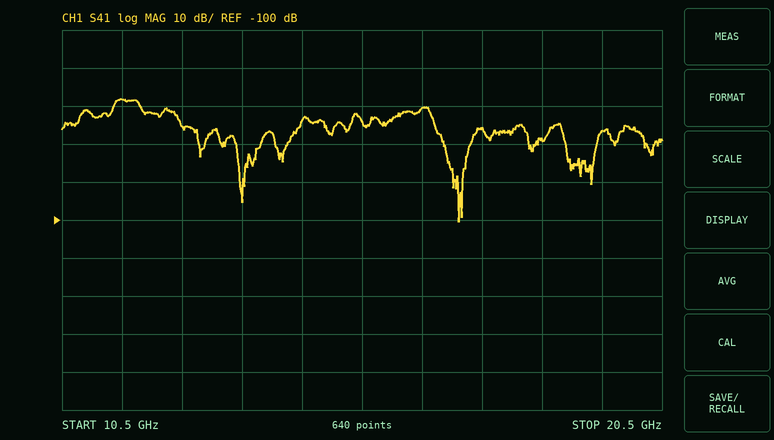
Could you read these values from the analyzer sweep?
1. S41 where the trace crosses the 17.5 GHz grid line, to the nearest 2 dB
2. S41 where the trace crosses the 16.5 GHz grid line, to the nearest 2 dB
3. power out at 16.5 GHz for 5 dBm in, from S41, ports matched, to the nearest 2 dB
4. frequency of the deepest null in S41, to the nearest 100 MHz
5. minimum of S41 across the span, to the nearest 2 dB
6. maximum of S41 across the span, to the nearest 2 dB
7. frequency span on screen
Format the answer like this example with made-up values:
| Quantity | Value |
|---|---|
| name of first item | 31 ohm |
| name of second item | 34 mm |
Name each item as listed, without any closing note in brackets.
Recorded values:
| Quantity | Value |
|---|---|
| S41 where the trace crosses the 17.5 GHz grid line, to the nearest 2 dB | -76 dB |
| S41 where the trace crosses the 16.5 GHz grid line, to the nearest 2 dB | -70 dB |
| power out at 16.5 GHz for 5 dBm in, from S41, ports matched, to the nearest 2 dB | -66 dBm |
| frequency of the deepest null in S41, to the nearest 100 MHz | 17.1 GHz |
| minimum of S41 across the span, to the nearest 2 dB | -100 dB |
| maximum of S41 across the span, to the nearest 2 dB | -68 dB |
| frequency span on screen | 10 GHz |
